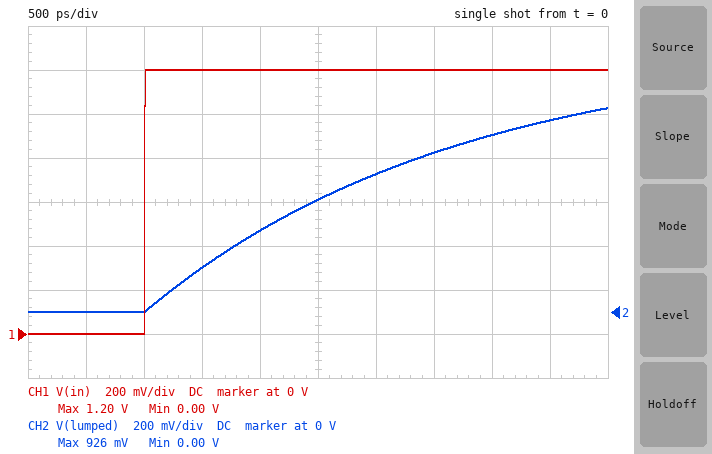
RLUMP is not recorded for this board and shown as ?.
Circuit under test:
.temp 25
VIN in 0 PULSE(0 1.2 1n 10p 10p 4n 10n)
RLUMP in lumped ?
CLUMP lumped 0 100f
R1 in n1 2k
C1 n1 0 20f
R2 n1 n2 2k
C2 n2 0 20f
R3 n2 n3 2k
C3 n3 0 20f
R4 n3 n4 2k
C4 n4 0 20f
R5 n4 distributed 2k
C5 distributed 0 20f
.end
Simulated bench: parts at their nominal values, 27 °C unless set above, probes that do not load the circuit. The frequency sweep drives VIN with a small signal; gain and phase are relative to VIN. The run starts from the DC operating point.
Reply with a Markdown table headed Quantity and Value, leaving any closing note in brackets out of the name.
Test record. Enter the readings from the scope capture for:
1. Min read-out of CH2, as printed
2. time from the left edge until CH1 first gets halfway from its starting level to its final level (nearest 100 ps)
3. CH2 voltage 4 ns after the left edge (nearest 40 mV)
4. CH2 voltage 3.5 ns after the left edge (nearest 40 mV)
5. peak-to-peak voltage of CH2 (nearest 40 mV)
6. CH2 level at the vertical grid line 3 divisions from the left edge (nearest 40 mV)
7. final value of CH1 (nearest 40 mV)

| Quantity | Value |
|---|---|
| Min read-out of CH2, as printed | 0.00 V |
| time from the left edge until CH1 first gets halfway from its starting level to its final level | 1.0 ns |
| CH2 voltage 4 ns after the left edge | 800 mV |
| CH2 voltage 3.5 ns after the left edge | 720 mV |
| peak-to-peak voltage of CH2 | 920 mV |
| CH2 level at the vertical grid line 3 divisions from the left edge | 200 mV |
| final value of CH1 | 1.20 V |
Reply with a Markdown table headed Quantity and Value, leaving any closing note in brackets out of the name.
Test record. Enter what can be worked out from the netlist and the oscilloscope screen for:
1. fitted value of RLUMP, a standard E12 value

| Quantity | Value |
|---|---|
| fitted value of RLUMP, a standard E12 value | 27 kΩ |
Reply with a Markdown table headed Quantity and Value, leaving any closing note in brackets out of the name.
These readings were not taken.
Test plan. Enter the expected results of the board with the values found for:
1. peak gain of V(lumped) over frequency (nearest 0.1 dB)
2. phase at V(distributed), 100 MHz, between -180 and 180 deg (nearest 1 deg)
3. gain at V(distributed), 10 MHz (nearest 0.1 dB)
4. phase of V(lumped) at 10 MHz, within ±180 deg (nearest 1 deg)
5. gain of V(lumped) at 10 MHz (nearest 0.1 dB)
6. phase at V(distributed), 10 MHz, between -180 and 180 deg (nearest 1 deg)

| Quantity | Value |
|---|---|
| peak gain of V(lumped) over frequency | 0 dB |
| phase at V(distributed), 100 MHz, between -180 and 180 deg | -21 deg |
| gain at V(distributed), 10 MHz | 0 dB |
| phase of V(lumped) at 10 MHz, within ±180 deg | -10 deg |
| gain of V(lumped) at 10 MHz | -0.1 dB |
| phase at V(distributed), 10 MHz, between -180 and 180 deg | -2 deg |
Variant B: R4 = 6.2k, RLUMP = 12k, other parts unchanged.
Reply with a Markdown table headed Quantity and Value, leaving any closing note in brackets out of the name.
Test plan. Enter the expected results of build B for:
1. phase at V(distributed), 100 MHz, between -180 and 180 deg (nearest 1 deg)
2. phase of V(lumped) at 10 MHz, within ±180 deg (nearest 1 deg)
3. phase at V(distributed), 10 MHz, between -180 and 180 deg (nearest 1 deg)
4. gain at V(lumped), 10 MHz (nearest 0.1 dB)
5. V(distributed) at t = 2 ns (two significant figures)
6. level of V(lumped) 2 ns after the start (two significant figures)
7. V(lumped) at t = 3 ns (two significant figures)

| Quantity | Value |
|---|---|
| phase at V(distributed), 100 MHz, between -180 and 180 deg | -27 deg |
| phase of V(lumped) at 10 MHz, within ±180 deg | -4 deg |
| phase at V(distributed), 10 MHz, between -180 and 180 deg | -3 deg |
| gain at V(lumped), 10 MHz | 0 dB |
| V(distributed) at t = 2 ns | 890 mV |
| level of V(lumped) 2 ns after the start | 680 mV |
| V(lumped) at t = 3 ns | 970 mV |
